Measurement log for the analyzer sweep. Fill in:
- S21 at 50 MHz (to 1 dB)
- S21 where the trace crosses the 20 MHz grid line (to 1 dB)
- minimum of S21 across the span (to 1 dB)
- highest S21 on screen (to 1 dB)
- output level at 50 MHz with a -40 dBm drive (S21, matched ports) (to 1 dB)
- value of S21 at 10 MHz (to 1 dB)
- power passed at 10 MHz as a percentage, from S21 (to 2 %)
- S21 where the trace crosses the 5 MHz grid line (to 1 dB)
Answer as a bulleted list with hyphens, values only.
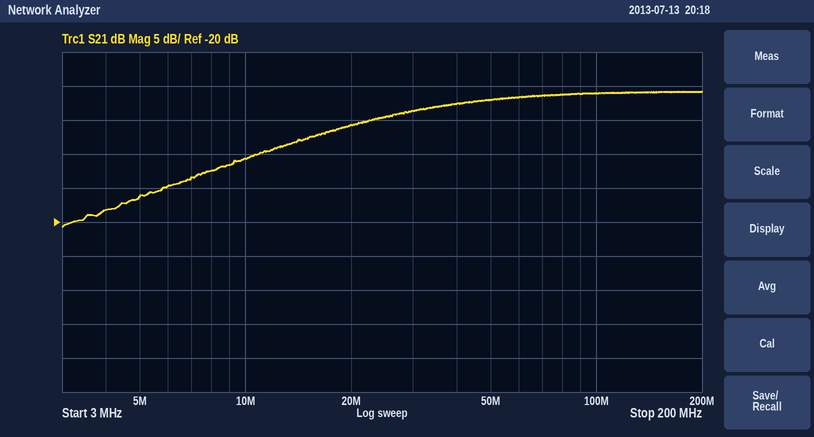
- -2 dB
- -6 dB
- -21 dB
- -1 dB
- -42 dBm
- -11 dB
- 8 %
- -16 dB
